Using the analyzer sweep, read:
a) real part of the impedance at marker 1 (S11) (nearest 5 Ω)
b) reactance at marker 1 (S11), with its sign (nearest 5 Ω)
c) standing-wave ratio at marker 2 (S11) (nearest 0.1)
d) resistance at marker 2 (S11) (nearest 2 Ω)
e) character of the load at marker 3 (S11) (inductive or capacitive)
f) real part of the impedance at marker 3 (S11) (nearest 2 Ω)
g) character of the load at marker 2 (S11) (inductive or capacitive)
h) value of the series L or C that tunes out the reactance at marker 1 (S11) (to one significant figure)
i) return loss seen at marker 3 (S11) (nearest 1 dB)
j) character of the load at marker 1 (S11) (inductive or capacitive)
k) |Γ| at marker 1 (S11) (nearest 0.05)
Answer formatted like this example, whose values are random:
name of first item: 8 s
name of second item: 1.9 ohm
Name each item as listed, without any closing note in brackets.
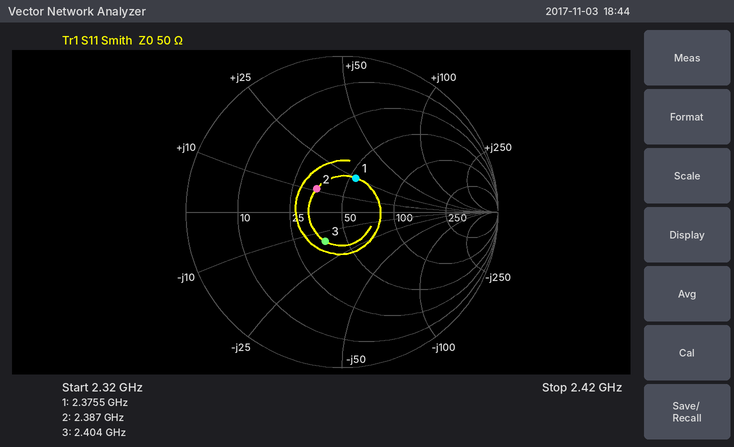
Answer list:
real part of the impedance at marker 1 (S11): 55 Ω
reactance at marker 1 (S11), with its sign: +25 Ω
standing-wave ratio at marker 2 (S11): 1.6
resistance at marker 2 (S11): 34 Ω
character of the load at marker 3 (S11): capacitive
real part of the impedance at marker 3 (S11): 38 Ω
character of the load at marker 2 (S11): inductive
value of the series L or C that tunes out the reactance at marker 1 (S11): 3 pF
return loss seen at marker 3 (S11): 13 dB
character of the load at marker 1 (S11): inductive
|Γ| at marker 1 (S11): 0.25
